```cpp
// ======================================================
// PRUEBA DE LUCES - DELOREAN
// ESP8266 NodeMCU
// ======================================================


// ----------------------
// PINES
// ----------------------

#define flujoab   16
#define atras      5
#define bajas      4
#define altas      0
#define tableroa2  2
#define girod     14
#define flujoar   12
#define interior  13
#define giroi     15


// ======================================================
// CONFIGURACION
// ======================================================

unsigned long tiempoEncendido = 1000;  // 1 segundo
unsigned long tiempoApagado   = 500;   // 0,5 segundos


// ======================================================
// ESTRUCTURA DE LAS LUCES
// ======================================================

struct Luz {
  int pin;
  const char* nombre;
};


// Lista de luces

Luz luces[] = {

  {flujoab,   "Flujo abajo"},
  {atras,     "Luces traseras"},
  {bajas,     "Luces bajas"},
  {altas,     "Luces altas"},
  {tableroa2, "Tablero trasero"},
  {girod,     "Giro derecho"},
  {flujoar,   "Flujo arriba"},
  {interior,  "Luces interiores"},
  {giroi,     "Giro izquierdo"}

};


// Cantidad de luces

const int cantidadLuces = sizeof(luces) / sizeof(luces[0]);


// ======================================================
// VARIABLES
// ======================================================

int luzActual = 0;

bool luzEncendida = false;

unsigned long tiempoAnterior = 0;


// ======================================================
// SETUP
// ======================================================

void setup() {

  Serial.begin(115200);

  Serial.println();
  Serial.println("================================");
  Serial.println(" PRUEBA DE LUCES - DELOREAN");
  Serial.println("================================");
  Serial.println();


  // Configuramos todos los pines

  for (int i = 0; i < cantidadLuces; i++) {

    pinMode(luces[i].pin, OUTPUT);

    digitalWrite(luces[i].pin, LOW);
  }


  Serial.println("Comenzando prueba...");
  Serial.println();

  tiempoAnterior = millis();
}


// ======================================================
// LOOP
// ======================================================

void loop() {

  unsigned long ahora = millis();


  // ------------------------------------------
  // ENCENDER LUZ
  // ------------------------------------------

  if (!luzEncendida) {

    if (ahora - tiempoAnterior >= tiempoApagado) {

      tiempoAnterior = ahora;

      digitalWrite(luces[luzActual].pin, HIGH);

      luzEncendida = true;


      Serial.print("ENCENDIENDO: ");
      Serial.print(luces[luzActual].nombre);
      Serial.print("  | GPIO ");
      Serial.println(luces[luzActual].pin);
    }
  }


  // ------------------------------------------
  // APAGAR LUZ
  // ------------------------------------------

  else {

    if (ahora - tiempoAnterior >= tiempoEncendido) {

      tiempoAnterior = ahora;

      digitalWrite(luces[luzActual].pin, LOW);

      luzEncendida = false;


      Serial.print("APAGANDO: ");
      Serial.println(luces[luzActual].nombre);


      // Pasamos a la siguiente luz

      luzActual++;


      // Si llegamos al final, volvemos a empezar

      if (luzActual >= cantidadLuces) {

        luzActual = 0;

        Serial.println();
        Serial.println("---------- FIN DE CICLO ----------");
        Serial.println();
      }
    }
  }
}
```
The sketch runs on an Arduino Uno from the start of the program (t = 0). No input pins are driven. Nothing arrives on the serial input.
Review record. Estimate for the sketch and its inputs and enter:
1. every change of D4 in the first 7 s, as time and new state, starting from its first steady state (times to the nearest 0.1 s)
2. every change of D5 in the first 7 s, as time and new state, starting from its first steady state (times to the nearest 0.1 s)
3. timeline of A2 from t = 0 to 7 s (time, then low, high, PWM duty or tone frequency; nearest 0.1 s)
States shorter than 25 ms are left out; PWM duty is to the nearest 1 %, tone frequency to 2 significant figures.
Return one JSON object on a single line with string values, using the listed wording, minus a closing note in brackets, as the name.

{"every change of D4 in the first 7 s, as time and new state, starting from its first steady state": "0 s low; 3.5 s high; 4.5 s low", "every change of D5 in the first 7 s, as time and new state, starting from its first steady state": "0 s low; 2 s high; 3 s low", "timeline of A2 from t = 0 to 7 s": "0 s low; 0.5 s high; 1.5 s low"}
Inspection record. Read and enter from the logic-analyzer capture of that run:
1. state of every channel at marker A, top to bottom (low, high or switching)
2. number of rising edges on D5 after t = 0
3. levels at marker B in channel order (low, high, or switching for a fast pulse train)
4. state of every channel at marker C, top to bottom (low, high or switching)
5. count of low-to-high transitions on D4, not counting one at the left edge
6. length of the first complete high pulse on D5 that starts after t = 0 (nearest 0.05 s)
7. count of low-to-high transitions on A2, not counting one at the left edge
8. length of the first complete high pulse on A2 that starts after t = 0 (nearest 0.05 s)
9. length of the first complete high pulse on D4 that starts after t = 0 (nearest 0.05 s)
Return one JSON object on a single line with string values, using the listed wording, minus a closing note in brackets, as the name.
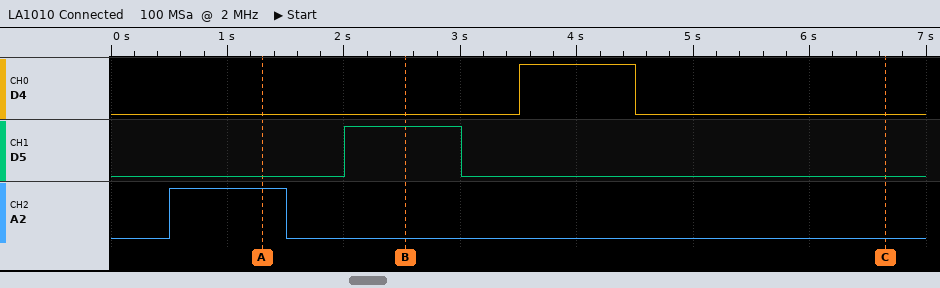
{"state of every channel at marker A, top to bottom": "D4 low, D5 low, A2 high", "number of rising edges on D5 after t = 0": "1", "levels at marker B in channel order": "D4 low, D5 high, A2 low", "state of every channel at marker C, top to bottom": "D4 low, D5 low, A2 low", "count of low-to-high transitions on D4, not counting one at the left edge": "1", "length of the first complete high pulse on D5 that starts after t = 0": "1.00 s", "count of low-to-high transitions on A2, not counting one at the left edge": "1", "length of the first complete high pulse on A2 that starts after t = 0": "1.00 s", "length of the first complete high pulse on D4 that starts after t = 0": "1.00 s"}
